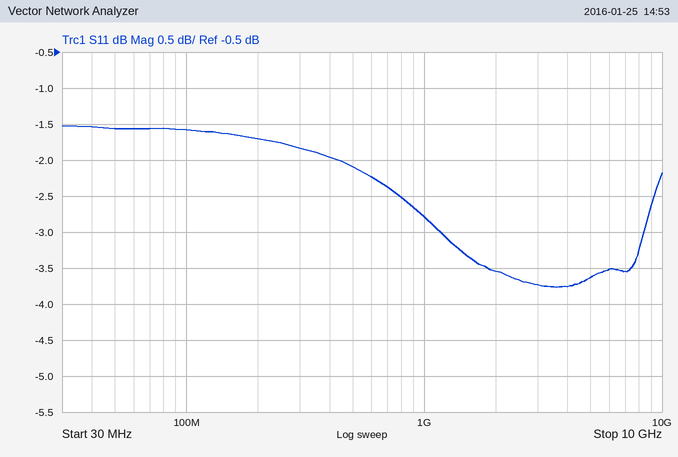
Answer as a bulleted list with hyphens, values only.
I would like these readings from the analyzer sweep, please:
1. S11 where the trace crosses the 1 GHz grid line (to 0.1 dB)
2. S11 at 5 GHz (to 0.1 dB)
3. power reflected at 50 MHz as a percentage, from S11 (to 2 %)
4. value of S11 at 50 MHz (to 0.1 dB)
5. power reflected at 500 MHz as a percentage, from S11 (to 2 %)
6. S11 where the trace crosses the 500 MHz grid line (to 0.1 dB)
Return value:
- -2.8 dB
- -3.6 dB
- 70 %
- -1.6 dB
- 62 %
- -2.1 dB
